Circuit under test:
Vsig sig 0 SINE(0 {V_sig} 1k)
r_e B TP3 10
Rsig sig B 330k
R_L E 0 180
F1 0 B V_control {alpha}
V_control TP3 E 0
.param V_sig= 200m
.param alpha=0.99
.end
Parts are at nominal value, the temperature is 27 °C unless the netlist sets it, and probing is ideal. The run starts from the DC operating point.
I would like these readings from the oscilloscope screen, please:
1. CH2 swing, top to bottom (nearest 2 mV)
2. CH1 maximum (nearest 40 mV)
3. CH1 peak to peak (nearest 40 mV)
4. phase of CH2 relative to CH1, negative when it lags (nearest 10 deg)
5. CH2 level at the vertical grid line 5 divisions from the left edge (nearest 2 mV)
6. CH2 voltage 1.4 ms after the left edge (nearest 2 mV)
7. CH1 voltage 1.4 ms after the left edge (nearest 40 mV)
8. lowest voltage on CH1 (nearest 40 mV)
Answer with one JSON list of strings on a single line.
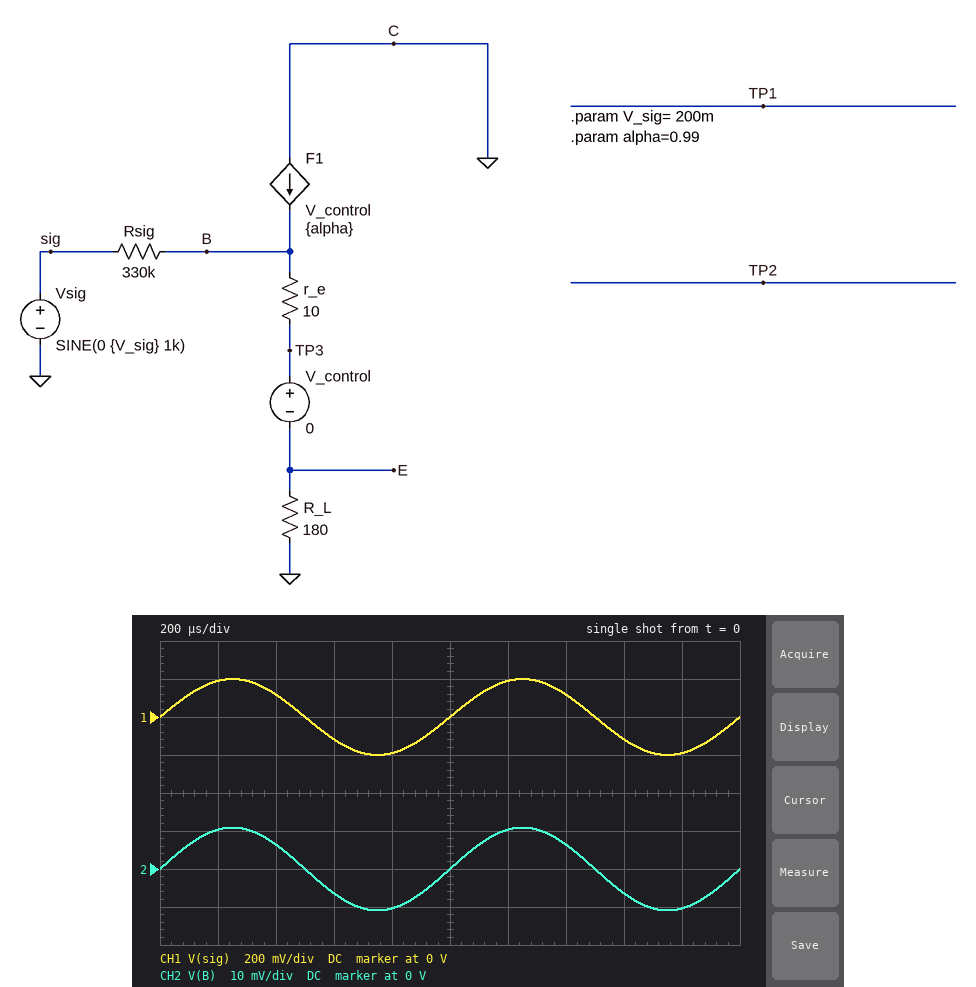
["22 mV", "200 mV", "400 mV", "0 deg", "0 V", "6 mV", "120 mV", "-200 mV"]
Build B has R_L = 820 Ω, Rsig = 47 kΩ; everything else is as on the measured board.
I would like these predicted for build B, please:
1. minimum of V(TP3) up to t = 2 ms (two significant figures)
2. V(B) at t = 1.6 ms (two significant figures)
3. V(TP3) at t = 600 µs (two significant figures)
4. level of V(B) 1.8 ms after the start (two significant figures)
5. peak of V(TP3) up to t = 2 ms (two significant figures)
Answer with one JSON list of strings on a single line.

["-130 mV", "-75 mV", "-74 mV", "-120 mV", "130 mV"]
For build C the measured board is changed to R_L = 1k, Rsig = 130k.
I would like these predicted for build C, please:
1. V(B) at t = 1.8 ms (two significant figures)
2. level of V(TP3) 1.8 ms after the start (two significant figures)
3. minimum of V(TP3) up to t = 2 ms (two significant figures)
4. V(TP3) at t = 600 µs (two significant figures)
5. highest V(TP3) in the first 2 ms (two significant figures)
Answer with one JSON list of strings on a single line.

["-83 mV", "-82 mV", "-87 mV", "-51 mV", "87 mV"]
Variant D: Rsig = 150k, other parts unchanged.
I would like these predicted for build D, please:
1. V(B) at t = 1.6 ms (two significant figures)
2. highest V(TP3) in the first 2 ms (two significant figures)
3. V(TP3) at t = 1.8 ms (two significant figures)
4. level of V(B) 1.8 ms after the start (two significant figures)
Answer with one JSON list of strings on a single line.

["-13 mV", "21 mV", "-20 mV", "-21 mV"]
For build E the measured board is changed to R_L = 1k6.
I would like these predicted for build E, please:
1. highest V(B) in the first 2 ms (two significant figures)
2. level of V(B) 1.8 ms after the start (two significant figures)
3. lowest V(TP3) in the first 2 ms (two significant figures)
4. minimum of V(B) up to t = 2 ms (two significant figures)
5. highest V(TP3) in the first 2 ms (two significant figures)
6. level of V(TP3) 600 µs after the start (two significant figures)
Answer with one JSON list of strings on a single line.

["66 mV", "-62 mV", "-65 mV", "-66 mV", "65 mV", "-38 mV"]
